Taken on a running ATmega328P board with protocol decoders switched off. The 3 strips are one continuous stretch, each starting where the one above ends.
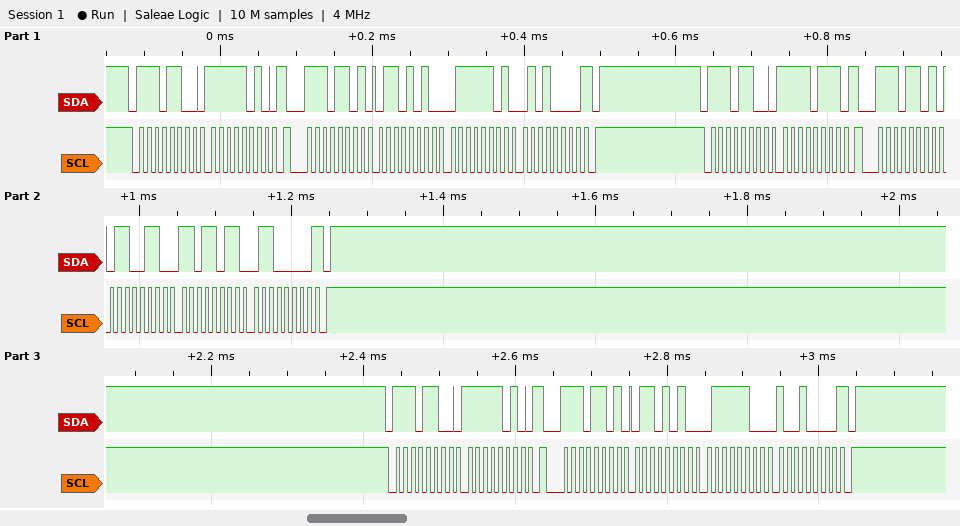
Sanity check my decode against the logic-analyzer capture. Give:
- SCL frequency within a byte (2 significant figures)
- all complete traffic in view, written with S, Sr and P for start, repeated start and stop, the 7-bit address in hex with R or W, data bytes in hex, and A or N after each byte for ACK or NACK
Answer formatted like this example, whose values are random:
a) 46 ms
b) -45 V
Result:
a) 100 kHz
b) S 76W A FA A Sr 76R A 6A A 7D A 50 N P S 76W A F7 A Sr 76R A 66 A DB A 60 N P S 76W A FA A Sr 76R A 6A A 7C A 90 N P
